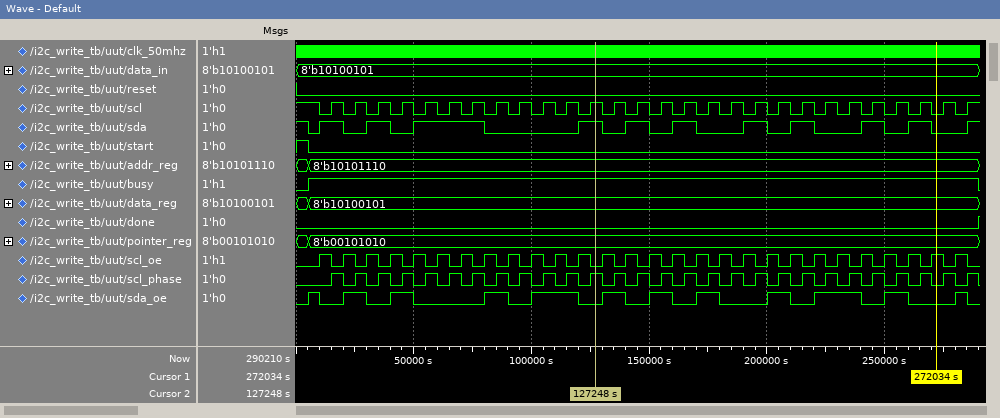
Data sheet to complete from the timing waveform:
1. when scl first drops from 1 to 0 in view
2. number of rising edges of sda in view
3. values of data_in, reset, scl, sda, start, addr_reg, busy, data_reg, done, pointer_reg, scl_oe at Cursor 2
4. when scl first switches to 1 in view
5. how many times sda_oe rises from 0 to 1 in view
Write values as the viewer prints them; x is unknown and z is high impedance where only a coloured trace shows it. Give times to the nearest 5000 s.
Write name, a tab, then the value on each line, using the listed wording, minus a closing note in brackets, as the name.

when scl first drops from 1 to 0 in view	10000 s
number of rising edges of sda in view	11
values of data_in, reset, scl, sda, start, addr_reg, busy, data_reg, done, pointer_reg, scl_oe at Cursor 2	data_in=8'b10100101, reset=0, scl=1, sda=1, start=0, addr_reg=8'b10101110, busy=1, data_reg=8'b10100101, done=0, pointer_reg=8'b00101010, scl_oe=0
when scl first switches to 1 in view	15000 s
how many times sda_oe rises from 0 to 1 in view	12
